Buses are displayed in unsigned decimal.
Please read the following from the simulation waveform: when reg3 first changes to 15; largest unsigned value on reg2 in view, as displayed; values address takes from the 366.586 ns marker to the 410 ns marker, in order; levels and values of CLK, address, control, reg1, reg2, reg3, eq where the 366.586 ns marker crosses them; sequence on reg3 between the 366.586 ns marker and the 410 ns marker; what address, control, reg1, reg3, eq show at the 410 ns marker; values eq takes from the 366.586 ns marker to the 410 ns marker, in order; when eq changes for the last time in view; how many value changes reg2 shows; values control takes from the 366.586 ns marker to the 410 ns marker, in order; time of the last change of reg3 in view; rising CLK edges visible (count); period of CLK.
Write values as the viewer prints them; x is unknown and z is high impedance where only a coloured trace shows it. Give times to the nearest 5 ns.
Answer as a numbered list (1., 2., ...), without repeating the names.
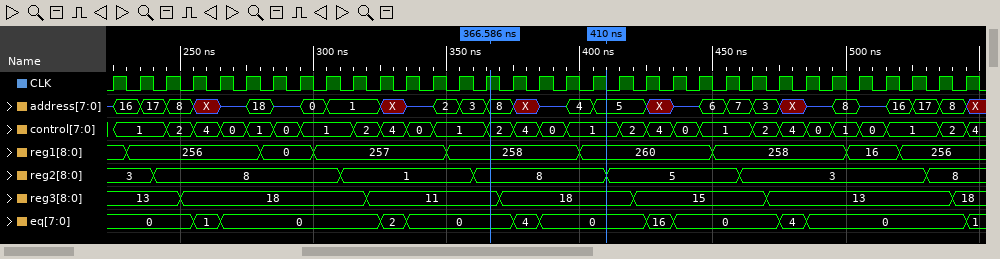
1. 420 ns
2. 8
3. 8, X, z, 4, 5
4. CLK=1, address=8, control=2, reg1=258, reg2=8, reg3=11, eq=0
5. 11, 18
6. address=5, control=1, reg1=260, reg3=18, eq=0
7. 0, 4, 0
8. 545 ns
9. 6
10. 2, 4, 0, 1
11. 540 ns
12. 33
13. 10 ns
